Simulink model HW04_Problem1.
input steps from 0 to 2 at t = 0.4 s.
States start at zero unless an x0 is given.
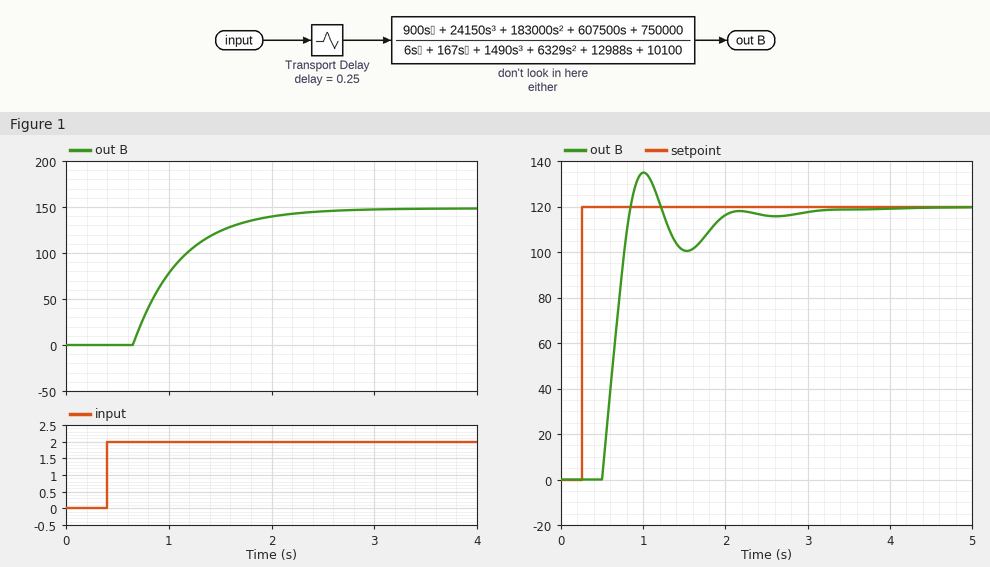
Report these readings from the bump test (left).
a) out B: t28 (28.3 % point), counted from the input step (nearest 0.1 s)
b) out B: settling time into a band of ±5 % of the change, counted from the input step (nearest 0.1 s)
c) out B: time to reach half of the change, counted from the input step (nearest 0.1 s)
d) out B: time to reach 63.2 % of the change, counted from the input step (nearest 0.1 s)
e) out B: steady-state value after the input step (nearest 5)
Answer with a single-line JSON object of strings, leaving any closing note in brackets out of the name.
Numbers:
{"out B: t28 (28.3 % point), counted from the input step": "0.4 s", "out B: settling time into a band of ±5 % of the change, counted from the input step": "1.7 s", "out B: time to reach half of the change, counted from the input step": "0.6 s", "out B: time to reach 63.2 % of the change, counted from the input step": "0.7 s", "out B: steady-state value after the input step": "150"}
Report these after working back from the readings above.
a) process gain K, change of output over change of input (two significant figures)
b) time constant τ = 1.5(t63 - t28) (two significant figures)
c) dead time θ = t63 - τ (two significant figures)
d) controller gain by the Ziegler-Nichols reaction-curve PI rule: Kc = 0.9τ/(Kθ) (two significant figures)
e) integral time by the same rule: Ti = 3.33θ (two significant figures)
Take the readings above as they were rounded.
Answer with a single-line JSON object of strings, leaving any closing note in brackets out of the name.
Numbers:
{"process gain K, change of output over change of input": "75", "time constant τ = 1.5(t63 - t28)": "0.45 s", "dead time θ = t63 - τ": "0.25 s", "controller gain by the Ziegler-Nichols reaction-curve PI rule: Kc = 0.9τ/(Kθ)": "0.022", "integral time by the same rule: Ti = 3.33θ": "0.83 s"}
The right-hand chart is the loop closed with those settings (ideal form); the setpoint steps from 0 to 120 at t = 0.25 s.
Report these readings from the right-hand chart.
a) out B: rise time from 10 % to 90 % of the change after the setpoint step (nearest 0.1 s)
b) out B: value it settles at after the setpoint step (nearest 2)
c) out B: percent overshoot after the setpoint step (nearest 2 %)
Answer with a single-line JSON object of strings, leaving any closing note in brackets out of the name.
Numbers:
{"out B: rise time from 10 % to 90 % of the change after the setpoint step": "0.3 s", "out B: value it settles at after the setpoint step": "120", "out B: percent overshoot after the setpoint step": "12 %"}
